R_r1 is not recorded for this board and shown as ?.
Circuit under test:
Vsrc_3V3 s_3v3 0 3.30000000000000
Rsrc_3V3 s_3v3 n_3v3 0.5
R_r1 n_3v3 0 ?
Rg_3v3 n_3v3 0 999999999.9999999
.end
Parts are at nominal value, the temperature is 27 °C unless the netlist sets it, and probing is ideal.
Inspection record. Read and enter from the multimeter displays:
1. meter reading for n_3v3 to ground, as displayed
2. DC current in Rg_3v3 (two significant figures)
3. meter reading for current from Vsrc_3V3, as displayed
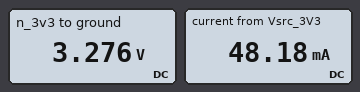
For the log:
3.276 V
3.3 nA
48.18 mA
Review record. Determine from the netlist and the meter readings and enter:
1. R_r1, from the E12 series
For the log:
68 Ω
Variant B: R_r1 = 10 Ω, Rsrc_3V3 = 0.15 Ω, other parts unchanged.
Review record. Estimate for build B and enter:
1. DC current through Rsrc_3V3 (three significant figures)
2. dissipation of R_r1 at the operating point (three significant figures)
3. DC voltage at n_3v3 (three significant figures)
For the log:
325 mA
1.06 W
3.25 V
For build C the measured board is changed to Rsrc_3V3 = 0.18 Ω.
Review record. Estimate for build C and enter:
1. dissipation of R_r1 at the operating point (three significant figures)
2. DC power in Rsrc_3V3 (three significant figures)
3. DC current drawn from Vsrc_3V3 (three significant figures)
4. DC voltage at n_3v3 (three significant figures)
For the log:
159 mW
422 µW
48.4 mA
3.29 V
